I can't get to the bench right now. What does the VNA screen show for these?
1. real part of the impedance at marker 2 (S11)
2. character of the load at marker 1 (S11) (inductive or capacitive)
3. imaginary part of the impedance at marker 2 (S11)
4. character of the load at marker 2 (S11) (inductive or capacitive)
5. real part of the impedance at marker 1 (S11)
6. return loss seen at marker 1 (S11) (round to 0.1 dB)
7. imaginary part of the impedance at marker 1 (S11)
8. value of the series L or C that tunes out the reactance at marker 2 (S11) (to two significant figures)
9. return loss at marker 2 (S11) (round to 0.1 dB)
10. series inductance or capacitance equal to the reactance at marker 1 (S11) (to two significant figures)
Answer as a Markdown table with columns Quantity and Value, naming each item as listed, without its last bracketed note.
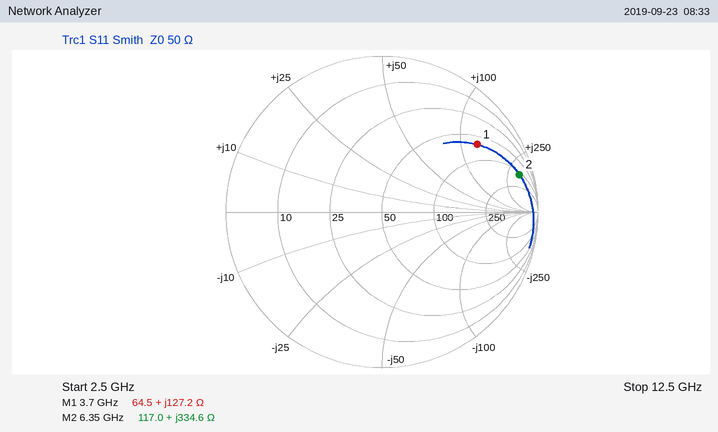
| Quantity | Value |
|---|---|
| real part of the impedance at marker 2 | 117.0 Ω |
| character of the load at marker 1 (S11) | inductive |
| imaginary part of the impedance at marker 2 | +334.6 Ω |
| character of the load at marker 2 (S11) | inductive |
| real part of the impedance at marker 1 | 64.5 Ω |
| return loss seen at marker 1 (S11) | 2.5 dB |
| imaginary part of the impedance at marker 1 | +127.2 Ω |
| value of the series L or C that tunes out the reactance at marker 2 (S11) | 75 fF |
| return loss at marker 2 (S11) | 0.8 dB |
| series inductance or capacitance equal to the reactance at marker 1 (S11) | 5.5 nH |
